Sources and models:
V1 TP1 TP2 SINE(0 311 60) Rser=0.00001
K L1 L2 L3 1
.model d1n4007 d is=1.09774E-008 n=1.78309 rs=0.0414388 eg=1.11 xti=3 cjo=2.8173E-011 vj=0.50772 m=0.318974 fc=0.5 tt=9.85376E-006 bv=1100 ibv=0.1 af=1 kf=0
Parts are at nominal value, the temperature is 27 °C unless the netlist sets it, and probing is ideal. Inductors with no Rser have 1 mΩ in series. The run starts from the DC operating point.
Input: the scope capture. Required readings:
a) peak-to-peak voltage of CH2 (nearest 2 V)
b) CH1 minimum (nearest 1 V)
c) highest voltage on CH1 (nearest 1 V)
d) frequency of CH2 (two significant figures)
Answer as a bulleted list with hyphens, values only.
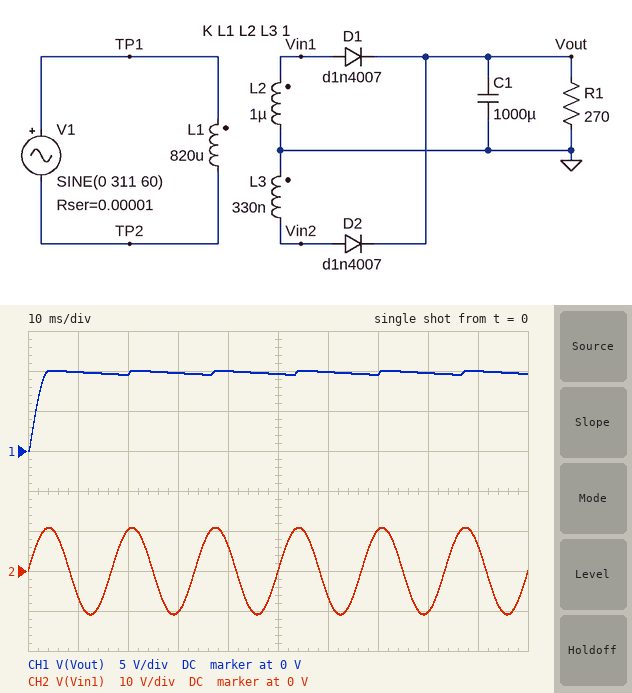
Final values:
- 22 V
- 0 V
- 10 V
- 60 Hz
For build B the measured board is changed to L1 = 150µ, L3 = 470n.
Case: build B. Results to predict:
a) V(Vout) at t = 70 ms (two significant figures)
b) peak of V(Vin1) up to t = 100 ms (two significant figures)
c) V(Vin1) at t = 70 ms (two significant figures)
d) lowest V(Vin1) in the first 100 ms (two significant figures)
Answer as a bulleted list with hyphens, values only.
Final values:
- 23 V
- 25 V
- 24 V
- -26 V
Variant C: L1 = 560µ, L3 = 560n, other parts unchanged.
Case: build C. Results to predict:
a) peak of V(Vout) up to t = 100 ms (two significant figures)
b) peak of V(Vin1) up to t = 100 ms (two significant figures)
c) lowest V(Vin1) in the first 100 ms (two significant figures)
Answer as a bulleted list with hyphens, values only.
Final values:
- 12 V
- 13 V
- -13 V
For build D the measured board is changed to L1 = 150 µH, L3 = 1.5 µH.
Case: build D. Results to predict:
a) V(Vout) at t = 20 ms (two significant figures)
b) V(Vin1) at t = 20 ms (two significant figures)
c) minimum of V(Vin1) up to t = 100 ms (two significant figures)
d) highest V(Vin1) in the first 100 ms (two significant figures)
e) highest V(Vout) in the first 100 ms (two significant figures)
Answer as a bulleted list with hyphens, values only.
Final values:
- 30 V
- 24 V
- -26 V
- 25 V
- 31 V
